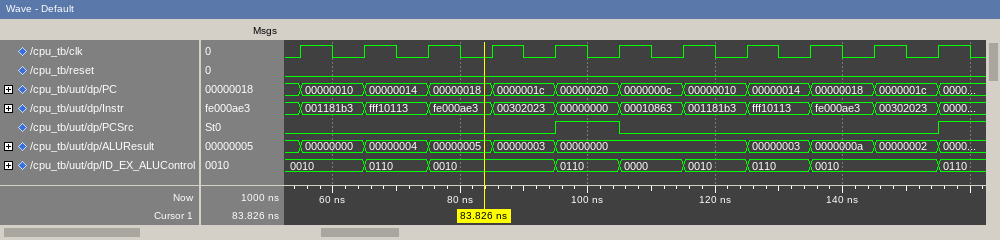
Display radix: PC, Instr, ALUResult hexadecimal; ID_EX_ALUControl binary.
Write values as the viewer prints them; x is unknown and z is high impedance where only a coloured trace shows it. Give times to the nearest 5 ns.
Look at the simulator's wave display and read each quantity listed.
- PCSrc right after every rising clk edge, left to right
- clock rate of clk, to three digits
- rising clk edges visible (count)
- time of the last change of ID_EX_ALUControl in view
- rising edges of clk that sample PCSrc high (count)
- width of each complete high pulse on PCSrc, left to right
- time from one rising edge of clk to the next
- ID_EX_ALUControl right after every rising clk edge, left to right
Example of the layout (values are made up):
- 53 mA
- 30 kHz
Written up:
- 0 0 0 0 1 0 0 0 0 0 1
- 100 MHz
- 11
- 155 ns
- 1
- 10 ns
- 10 ns
- 0010, 0110, 0010, 0010, 0110, 0000, 0010, 0110, 0010, 0010, 0110
